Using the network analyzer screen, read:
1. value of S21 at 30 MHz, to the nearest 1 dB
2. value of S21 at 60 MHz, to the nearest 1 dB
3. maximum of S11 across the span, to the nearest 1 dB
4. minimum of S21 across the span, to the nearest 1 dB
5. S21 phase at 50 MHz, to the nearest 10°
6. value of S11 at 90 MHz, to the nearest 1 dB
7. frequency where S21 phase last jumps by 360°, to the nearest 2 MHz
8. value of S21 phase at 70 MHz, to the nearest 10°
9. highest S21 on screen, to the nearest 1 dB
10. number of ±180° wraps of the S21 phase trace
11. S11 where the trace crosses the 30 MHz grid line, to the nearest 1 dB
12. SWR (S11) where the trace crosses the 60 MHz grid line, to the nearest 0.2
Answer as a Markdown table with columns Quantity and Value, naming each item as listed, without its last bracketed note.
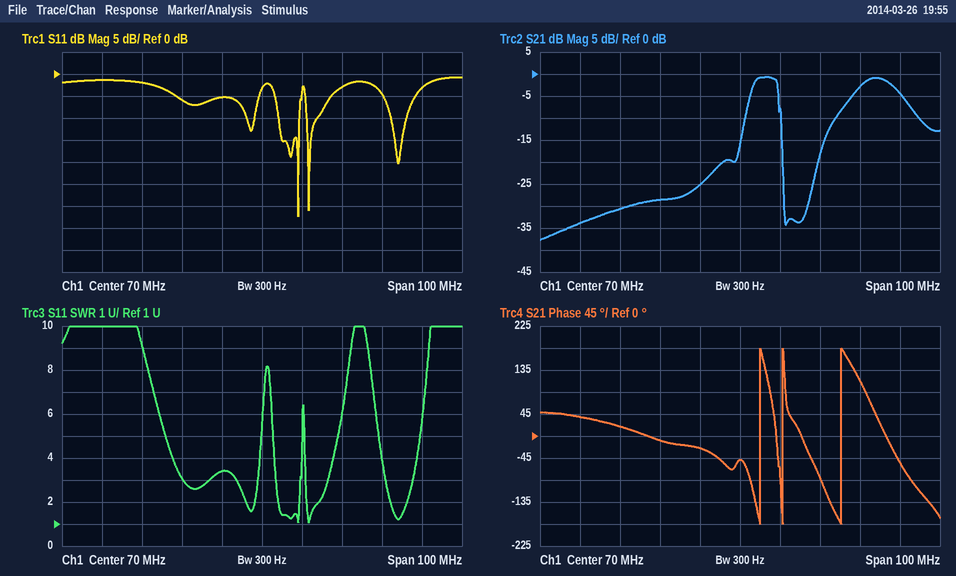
| Quantity | Value |
|---|---|
| value of S21 at 30 MHz, to the nearest 1 dB | -34 dB |
| value of S21 at 60 MHz, to the nearest 1 dB | -25 dB |
| maximum of S11 across the span, to the nearest 1 dB | -1 dB |
| minimum of S21 across the span, to the nearest 1 dB | -38 dB |
| S21 phase at 50 MHz, to the nearest 10° | -10° |
| value of S11 at 90 MHz, to the nearest 1 dB | -3 dB |
| frequency where S21 phase last jumps by 360°, to the nearest 2 MHz | 96 MHz |
| value of S21 phase at 70 MHz, to the nearest 10° | -50° |
| highest S21 on screen, to the nearest 1 dB | -1 dB |
| number of ±180° wraps of the S21 phase trace | 3 |
| S11 where the trace crosses the 30 MHz grid line, to the nearest 1 dB | -1 dB |
| SWR (S11) where the trace crosses the 60 MHz grid line, to the nearest 0.2 | 3.4 |
